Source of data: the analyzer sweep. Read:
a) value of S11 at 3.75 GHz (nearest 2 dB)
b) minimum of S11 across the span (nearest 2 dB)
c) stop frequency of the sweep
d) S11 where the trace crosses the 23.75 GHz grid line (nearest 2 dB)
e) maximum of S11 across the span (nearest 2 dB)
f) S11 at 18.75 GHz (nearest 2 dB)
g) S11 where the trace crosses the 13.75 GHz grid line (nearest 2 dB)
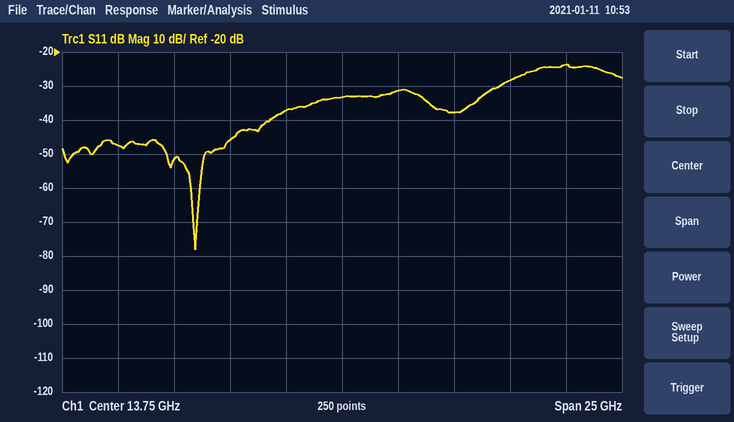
-48 dB
-78 dB
26.25 GHz
-24 dB
-24 dB
-38 dB
-34 dB
